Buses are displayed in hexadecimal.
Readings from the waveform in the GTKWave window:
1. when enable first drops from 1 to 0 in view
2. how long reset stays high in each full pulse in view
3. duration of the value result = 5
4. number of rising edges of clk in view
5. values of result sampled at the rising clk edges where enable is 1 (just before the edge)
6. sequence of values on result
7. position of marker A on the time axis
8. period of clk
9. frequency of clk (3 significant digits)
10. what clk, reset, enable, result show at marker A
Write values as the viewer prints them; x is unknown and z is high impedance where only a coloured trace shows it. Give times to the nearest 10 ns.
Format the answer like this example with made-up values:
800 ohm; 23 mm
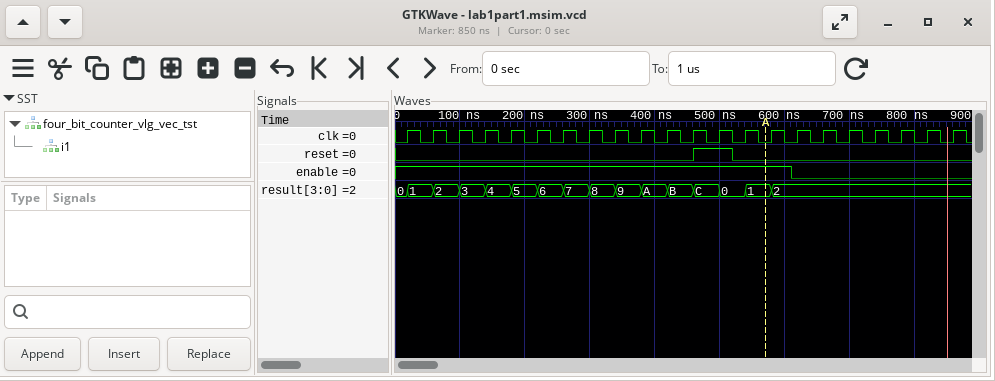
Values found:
610 ns; 60 ns; 40 ns; 22; 0, 1, 2, 3, 4, 5, 6, 7, 8, 9, A, B, C, 0, 1; 0, 1, 2, 3, 4, 5, 6, 7, 8, 9, A, B, C, 0, 1, 2; 570 ns; 40 ns; 25.0 MHz; clk=0, reset=0, enable=1, result=1
